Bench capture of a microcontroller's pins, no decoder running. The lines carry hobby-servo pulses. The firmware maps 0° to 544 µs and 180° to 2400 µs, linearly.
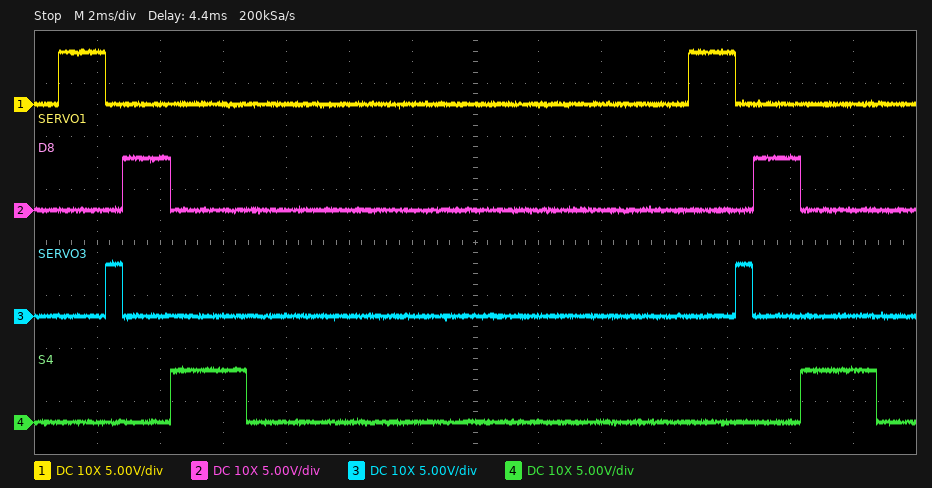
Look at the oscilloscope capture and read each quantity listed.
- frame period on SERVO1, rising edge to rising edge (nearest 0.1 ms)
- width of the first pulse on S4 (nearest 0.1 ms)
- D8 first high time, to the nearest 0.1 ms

20.0 ms
2.4 ms
1.5 ms
